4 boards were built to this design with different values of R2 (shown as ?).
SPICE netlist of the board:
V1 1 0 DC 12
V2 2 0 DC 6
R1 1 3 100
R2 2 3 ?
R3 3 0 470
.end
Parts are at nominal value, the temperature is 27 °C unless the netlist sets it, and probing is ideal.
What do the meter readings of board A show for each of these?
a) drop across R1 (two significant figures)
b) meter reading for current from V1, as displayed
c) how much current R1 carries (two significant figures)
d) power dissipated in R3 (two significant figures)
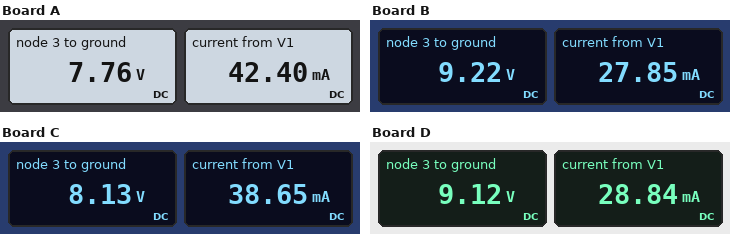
4.2 V
42.40 mA
42 mA
130 mW
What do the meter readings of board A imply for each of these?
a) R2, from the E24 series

68 Ω
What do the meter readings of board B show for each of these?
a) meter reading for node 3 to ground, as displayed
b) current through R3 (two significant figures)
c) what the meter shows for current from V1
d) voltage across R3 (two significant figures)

9.22 V
20 mA
27.85 mA
9.2 V
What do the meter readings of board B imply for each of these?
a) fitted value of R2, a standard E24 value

390 Ω
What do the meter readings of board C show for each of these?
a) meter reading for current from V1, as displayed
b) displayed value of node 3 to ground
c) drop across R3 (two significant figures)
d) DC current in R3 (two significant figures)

38.65 mA
8.13 V
8.1 V
17 mA
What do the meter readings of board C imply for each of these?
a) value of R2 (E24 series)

100 Ω
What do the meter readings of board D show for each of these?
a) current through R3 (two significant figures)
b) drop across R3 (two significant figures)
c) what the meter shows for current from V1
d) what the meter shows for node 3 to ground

19 mA
9.1 V
28.84 mA
9.12 V
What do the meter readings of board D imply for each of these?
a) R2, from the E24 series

330 Ω
